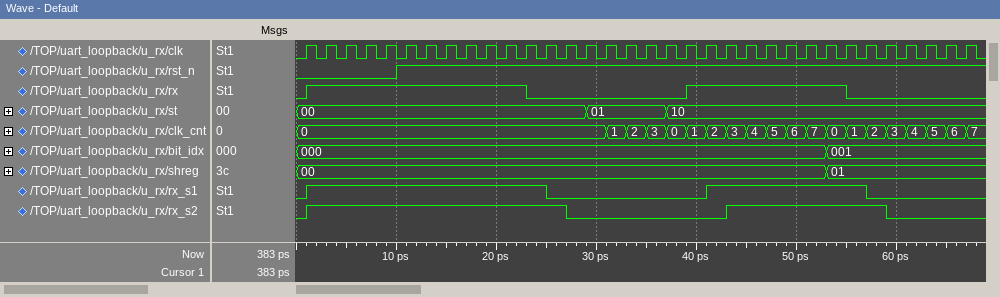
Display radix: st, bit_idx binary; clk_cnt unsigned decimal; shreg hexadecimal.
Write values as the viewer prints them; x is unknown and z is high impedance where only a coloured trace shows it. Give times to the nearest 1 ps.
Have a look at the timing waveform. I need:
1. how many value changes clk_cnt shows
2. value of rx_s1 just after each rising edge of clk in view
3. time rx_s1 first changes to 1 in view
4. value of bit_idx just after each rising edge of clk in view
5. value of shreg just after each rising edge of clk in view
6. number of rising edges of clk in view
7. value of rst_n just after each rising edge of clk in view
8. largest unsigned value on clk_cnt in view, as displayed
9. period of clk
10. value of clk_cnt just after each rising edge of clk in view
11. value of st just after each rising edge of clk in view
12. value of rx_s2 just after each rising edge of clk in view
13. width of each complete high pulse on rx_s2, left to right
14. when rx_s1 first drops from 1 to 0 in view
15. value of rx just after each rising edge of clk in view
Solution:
19
1 1 1 1 1 1 1 1 1 1 1 1 0 0 0 0 0 0 0 0 1 1 1 1 1 1 1 1 0 0 0 0 0 0
1 ps
000, 000, 000, 000, 000, 000, 000, 000, 000, 000, 000, 000, 000, 000, 000, 000, 000, 000, 000, 000, 000, 000, 000, 000, 000, 000, 001, 001, 001, 001, 001, 001, 001, 001
00, 00, 00, 00, 00, 00, 00, 00, 00, 00, 00, 00, 00, 00, 00, 00, 00, 00, 00, 00, 00, 00, 00, 00, 00, 00, 01, 01, 01, 01, 01, 01, 01, 01
34
0 0 0 0 0 1 1 1 1 1 1 1 1 1 1 1 1 1 1 1 1 1 1 1 1 1 1 1 1 1 1 1 1 1
7
2 ps
0, 0, 0, 0, 0, 0, 0, 0, 0, 0, 0, 0, 0, 0, 0, 1, 2, 3, 0, 1, 2, 3, 4, 5, 6, 7, 0, 1, 2, 3, 4, 5, 6, 7
00, 00, 00, 00, 00, 00, 00, 00, 00, 00, 00, 00, 00, 00, 01, 01, 01, 01, 10, 10, 10, 10, 10, 10, 10, 10, 10, 10, 10, 10, 10, 10, 10, 10
1 1 1 1 1 1 1 1 1 1 1 1 1 0 0 0 0 0 0 0 0 1 1 1 1 1 1 1 1 0 0 0 0 0
26 ps, 16 ps
25 ps
1 1 1 1 1 1 1 1 1 1 1 0 0 0 0 0 0 0 0 1 1 1 1 1 1 1 1 0 0 0 0 0 0 0
